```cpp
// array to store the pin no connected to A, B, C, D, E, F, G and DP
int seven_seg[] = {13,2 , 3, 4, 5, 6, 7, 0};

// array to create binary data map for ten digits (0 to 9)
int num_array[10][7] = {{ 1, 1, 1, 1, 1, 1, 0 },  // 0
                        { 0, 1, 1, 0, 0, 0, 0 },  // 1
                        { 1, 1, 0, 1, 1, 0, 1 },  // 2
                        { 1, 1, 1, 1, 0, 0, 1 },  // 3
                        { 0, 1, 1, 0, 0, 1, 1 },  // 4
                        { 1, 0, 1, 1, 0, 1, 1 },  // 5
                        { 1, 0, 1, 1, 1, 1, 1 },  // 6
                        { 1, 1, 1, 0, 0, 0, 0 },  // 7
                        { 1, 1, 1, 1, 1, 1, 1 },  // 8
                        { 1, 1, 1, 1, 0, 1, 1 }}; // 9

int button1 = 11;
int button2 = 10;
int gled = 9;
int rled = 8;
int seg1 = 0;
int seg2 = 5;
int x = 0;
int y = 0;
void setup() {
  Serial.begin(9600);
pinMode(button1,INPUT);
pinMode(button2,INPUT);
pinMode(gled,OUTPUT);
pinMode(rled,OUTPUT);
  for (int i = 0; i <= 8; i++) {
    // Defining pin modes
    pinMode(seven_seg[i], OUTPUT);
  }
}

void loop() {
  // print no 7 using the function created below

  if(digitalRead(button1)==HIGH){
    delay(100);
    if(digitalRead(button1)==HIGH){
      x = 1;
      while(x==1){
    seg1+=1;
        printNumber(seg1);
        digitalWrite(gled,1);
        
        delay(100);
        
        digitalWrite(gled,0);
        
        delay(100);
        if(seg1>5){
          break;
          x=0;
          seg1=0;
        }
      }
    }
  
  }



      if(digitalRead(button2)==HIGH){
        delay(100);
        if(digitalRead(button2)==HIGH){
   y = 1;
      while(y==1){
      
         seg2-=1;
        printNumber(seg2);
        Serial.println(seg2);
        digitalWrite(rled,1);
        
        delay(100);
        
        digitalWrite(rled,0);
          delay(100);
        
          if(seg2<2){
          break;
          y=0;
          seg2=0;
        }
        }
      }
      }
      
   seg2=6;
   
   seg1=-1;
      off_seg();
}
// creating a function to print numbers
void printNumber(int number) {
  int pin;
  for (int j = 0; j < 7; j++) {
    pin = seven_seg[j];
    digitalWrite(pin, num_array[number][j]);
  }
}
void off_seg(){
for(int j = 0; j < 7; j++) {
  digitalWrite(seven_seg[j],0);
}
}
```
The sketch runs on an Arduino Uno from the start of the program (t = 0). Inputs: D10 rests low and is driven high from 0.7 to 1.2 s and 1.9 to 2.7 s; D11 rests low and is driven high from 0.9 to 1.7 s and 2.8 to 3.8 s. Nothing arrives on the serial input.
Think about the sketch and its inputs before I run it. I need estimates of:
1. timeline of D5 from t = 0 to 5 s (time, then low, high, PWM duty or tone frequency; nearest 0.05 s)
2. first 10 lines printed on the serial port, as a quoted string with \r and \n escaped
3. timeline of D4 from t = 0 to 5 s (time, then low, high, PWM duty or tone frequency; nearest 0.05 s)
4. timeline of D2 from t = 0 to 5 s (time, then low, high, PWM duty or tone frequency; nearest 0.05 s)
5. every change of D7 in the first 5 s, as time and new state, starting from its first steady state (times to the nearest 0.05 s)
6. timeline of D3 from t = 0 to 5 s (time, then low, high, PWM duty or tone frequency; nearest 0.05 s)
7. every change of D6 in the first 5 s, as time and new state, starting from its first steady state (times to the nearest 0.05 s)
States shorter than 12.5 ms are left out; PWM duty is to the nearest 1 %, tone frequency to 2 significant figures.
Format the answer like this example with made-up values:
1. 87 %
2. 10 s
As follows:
1. 0 s low; 1.4 s high; 1.6 s low; 2.6 s high; 2.8 s low; 3.1 s high; 3.3 s low; 3.5 s high; 3.7 s low; 4.3 s high; 4.5 s low
2. "5\r\n4\r\n3\r\n2\r\n1\r\n5\r\n4\r\n3\r\n2\r\n1\r\n"
3. 0 s low; 0.8 s high; 1 s low; 1.2 s high; 1.6 s low; 2 s high; 2.2 s low; 2.4 s high; 2.8 s low; 3.1 s high; 3.3 s low; 3.5 s high; 3.9 s low; 4.1 s high; 4.5 s low
4. 0 s low; 1 s high; 1.8 s low; 2.2 s high; 3 s low; 3.1 s high; 4.1 s low
5. 0 s low; 0.8 s high; 1.6 s low; 2 s high; 2.8 s low; 3.5 s high; 4.5 s low
6. 0 s low; 0.8 s high; 1.4 s low; 1.6 s high; 1.8 s low; 2 s high; 2.6 s low; 2.8 s high; 3 s low; 3.1 s high; 3.5 s low; 3.7 s high; 4.5 s low
7. 0 s low; 0.8 s high; 1.2 s low; 2 s high; 2.4 s low; 3.1 s high; 3.3 s low; 3.9 s high; 4.5 s low
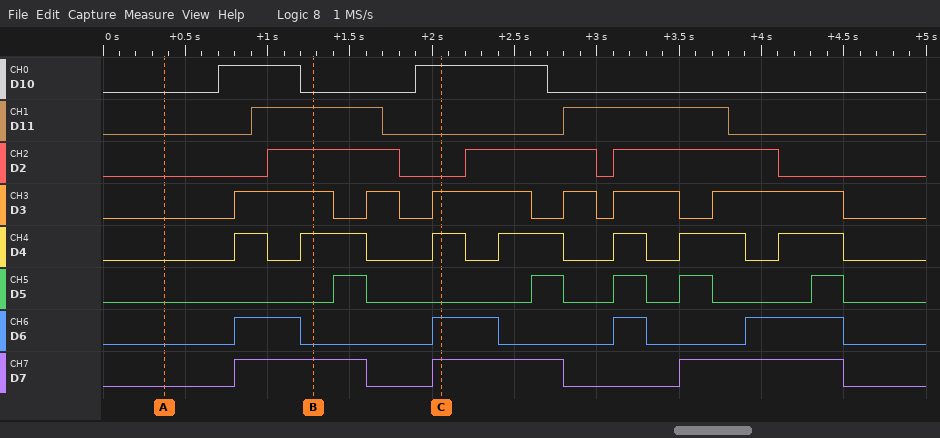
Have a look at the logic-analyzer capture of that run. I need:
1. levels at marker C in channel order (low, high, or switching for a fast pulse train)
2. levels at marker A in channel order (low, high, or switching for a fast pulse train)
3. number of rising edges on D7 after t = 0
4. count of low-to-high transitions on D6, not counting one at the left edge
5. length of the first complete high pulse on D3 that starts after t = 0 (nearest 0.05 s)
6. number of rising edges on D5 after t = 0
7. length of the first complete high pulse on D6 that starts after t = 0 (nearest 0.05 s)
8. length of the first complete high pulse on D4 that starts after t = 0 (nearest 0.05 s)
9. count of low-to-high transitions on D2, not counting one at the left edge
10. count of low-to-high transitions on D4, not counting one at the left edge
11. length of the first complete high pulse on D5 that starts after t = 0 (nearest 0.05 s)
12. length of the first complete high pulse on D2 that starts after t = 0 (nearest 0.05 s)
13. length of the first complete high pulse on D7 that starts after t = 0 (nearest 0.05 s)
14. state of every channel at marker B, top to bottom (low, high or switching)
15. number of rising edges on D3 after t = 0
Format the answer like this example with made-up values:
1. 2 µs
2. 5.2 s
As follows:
1. D10 high, D11 low, D2 low, D3 high, D4 high, D5 low, D6 high, D7 high
2. D10 low, D11 low, D2 low, D3 low, D4 low, D5 low, D6 low, D7 low
3. 3
4. 4
5. 0.60 s
6. 5
7. 0.40 s
8. 0.20 s
9. 3
10. 7
11. 0.20 s
12. 0.80 s
13. 0.80 s
14. D10 low, D11 high, D2 high, D3 high, D4 high, D5 low, D6 low, D7 high
15. 6
